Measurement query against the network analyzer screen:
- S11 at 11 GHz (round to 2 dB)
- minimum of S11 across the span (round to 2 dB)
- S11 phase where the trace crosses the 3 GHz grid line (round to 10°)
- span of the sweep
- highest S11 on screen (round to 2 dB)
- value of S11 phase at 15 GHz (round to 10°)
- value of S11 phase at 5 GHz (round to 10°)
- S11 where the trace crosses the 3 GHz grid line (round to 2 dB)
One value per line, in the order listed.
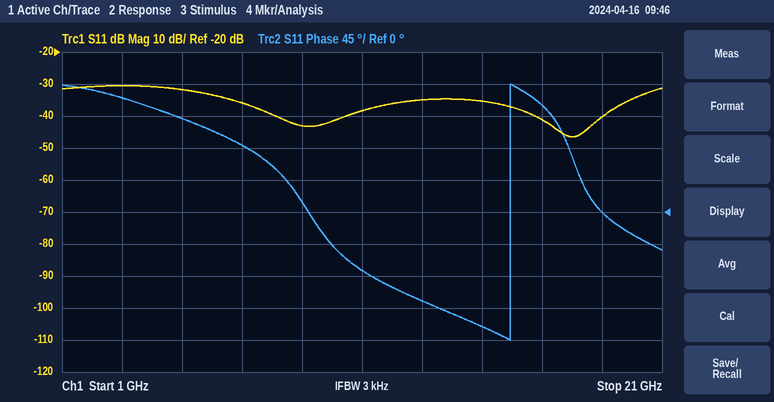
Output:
-38 dB
-46 dB
160°
20 GHz
-30 dB
-160°
130°
-30 dB
